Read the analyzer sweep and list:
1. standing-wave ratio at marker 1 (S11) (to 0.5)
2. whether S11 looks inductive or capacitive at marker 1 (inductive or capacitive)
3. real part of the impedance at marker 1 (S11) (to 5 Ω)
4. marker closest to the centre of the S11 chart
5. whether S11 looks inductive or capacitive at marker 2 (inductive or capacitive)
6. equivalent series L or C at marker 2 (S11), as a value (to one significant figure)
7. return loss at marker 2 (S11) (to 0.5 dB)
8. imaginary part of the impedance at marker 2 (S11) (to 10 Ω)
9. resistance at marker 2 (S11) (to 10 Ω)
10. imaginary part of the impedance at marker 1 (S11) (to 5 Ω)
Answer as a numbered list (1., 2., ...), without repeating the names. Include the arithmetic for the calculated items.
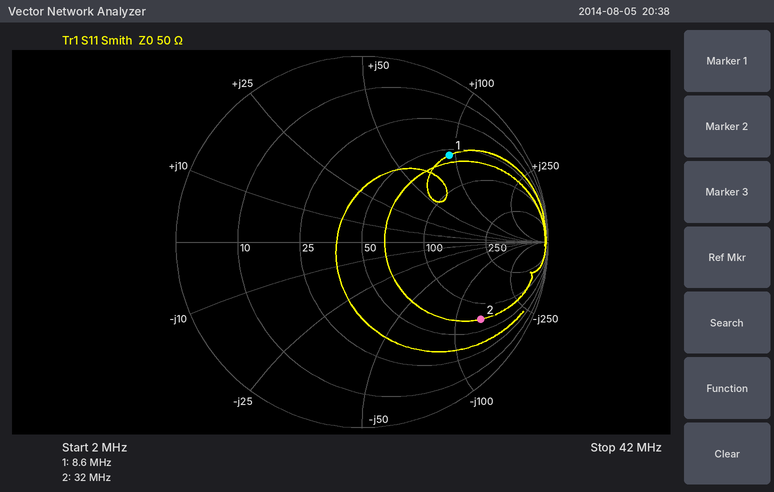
1. 5.0
2. inductive
3. 55 Ω
4. marker 1
5. capacitive
6. C = 1/(2π × 32 MHz × 140 Ω) ≈ 35.5 pF, so 40 pF to one significant figure
7. 2.5 dB
8. -140 Ω
9. 70 Ω
10. +95 Ω
